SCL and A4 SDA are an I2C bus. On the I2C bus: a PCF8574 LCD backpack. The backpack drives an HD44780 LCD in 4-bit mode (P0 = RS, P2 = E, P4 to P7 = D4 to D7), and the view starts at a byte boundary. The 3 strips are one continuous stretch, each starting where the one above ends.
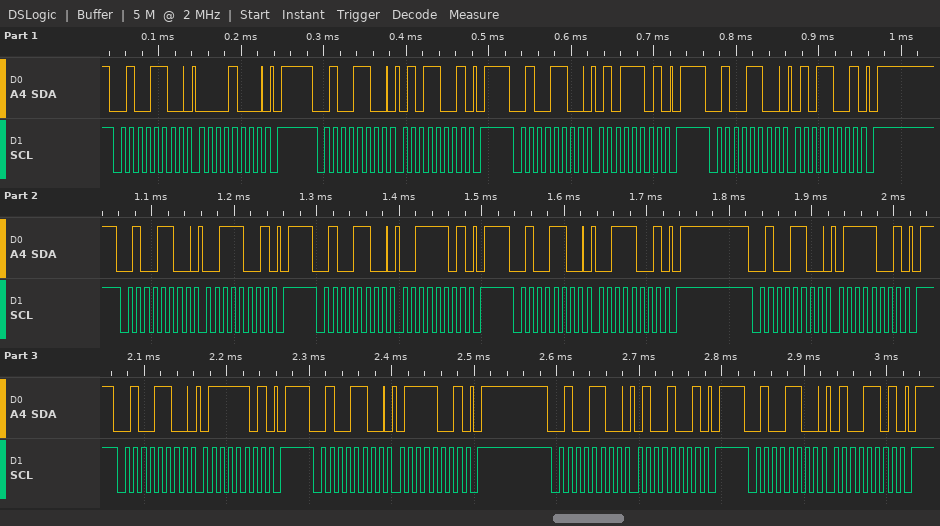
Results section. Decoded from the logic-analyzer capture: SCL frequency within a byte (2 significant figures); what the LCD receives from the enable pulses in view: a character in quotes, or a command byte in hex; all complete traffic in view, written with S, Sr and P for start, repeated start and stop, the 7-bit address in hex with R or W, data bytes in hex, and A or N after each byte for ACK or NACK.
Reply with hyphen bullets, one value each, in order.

- 100 kHz
- 'S'
- S 26W A 08 A P S 26W A 59 A P S 26W A 5D A P S 26W A 59 A P S 26W A 39 A P S 26W A 3D A P S 26W A 39 A P S 26W A 79 A P S 26W A 7D A P S 26W A 79 A P S 26W A 49 A P S 26W A 4D A P
